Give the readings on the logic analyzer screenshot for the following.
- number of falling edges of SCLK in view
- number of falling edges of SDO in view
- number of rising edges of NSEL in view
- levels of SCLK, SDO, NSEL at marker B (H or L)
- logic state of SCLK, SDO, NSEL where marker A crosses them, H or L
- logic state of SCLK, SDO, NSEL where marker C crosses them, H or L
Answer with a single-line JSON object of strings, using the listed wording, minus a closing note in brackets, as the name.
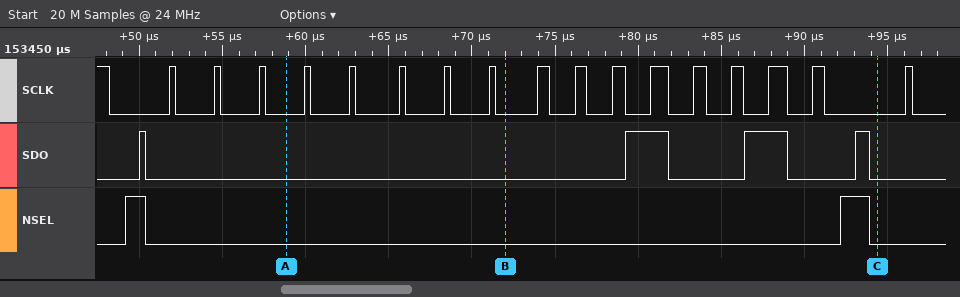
{"number of falling edges of SCLK in view": "18", "number of falling edges of SDO in view": "4", "number of rising edges of NSEL in view": "2", "levels of SCLK, SDO, NSEL at marker B": "SCLK=L, SDO=L, NSEL=L", "logic state of SCLK, SDO, NSEL where marker A crosses them, H or L": "SCLK=L, SDO=L, NSEL=L", "logic state of SCLK, SDO, NSEL where marker C crosses them, H or L": "SCLK=L, SDO=L, NSEL=L"}
